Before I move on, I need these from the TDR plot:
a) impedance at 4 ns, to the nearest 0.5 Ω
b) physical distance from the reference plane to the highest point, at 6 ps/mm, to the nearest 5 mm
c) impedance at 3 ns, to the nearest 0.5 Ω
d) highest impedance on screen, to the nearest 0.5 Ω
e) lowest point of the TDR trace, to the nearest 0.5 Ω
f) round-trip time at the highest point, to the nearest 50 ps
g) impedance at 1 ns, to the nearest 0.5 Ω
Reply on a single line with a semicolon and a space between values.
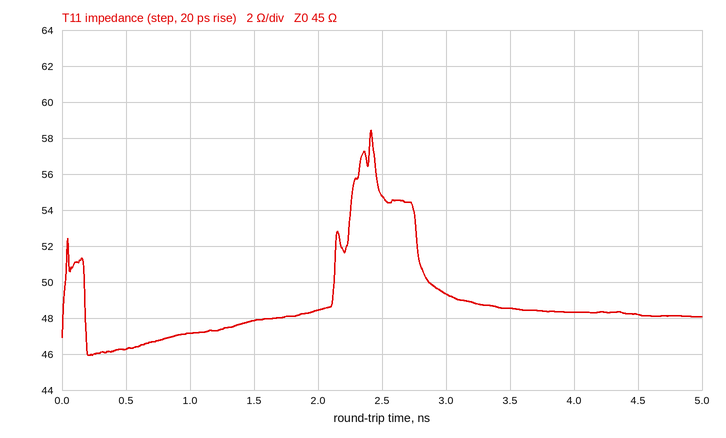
48.5 Ω; 200 mm; 49.5 Ω; 58.5 Ω; 46.0 Ω; 2.40 ns; 47.0 Ω
